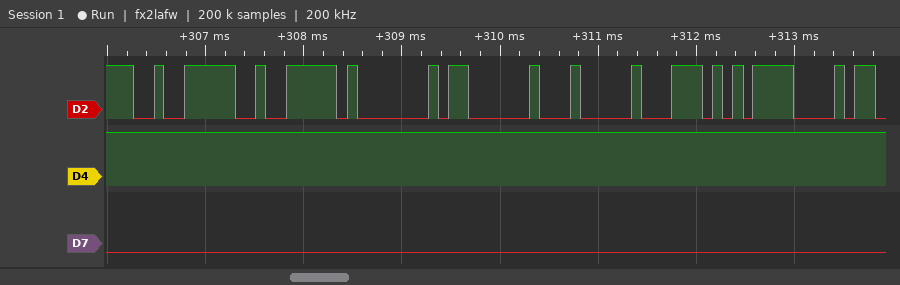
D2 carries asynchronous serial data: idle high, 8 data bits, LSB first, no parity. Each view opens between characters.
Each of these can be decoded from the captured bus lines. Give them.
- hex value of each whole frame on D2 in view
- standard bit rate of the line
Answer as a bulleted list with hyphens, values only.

- F2, F2, 01, 03, 04, 5C, 0F
- 9600 baud
